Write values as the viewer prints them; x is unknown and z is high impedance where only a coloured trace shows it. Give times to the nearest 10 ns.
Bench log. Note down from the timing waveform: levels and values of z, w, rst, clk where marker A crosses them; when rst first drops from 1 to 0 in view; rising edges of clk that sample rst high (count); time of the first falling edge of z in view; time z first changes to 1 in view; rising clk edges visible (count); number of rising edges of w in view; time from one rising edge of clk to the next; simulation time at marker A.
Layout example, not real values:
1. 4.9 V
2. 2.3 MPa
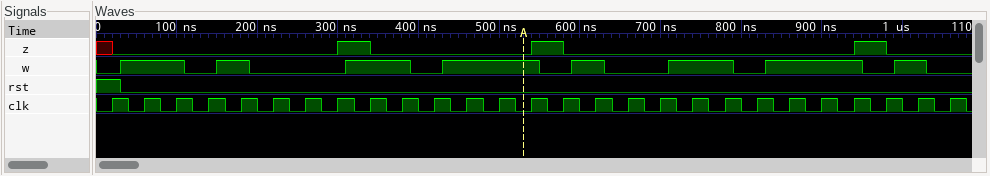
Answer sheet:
1. z=0, w=1, rst=0, clk=0
2. 30 ns
3. 1
4. 340 ns
5. 300 ns
6. 27
7. 8
8. 40 ns
9. 530 ns
